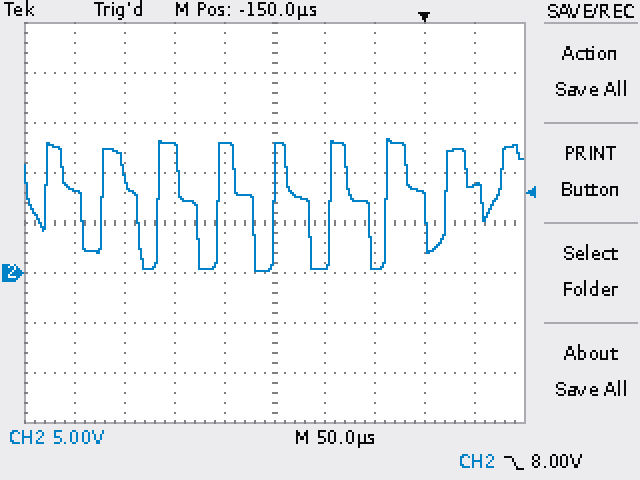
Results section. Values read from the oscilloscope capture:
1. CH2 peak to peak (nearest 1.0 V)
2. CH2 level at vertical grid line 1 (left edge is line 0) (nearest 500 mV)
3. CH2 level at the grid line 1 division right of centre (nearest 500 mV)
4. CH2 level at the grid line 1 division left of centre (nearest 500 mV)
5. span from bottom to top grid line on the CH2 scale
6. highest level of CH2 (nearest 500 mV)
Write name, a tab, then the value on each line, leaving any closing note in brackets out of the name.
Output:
CH2 peak to peak	13.0 V
CH2 level at vertical grid line 1 (left edge is line 0)	8.5 V
CH2 level at the grid line 1 division right of centre	500 mV
CH2 level at the grid line 1 division left of centre	13.0 V
span from bottom to top grid line on the CH2 scale	40 V
highest level of CH2	13.5 V
